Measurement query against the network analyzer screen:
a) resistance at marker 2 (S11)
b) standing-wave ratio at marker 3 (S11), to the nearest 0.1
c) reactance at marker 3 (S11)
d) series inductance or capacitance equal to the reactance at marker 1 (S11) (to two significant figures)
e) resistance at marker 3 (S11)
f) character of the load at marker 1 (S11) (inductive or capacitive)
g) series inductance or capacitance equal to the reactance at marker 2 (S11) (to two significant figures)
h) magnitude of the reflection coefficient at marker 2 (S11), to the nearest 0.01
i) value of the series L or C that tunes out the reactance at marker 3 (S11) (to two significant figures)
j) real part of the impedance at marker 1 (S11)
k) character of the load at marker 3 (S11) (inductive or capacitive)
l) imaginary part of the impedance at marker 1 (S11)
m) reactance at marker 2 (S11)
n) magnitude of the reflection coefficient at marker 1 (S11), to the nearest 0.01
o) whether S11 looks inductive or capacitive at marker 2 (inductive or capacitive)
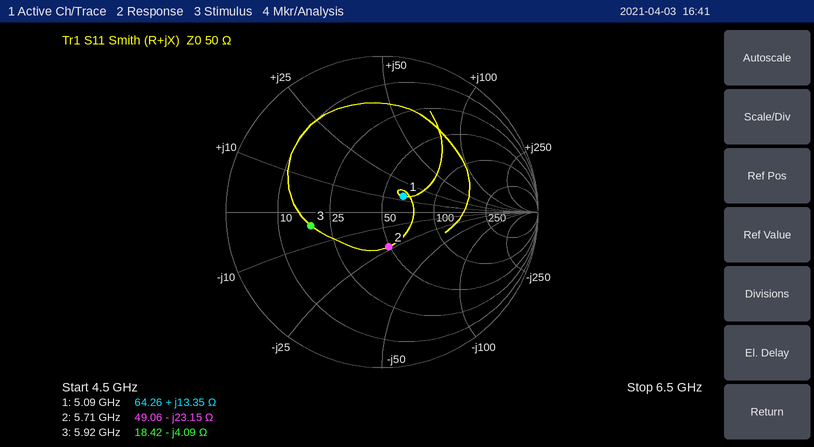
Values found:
49.06 Ω
2.7
-4.09 Ω
420 pH
18.42 Ω
inductive
1.2 pF
0.23
110 pH
64.26 Ω
capacitive
+13.35 Ω
-23.15 Ω
0.17
capacitive
